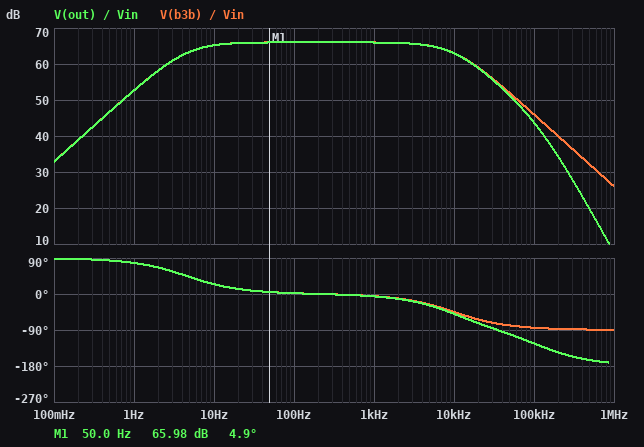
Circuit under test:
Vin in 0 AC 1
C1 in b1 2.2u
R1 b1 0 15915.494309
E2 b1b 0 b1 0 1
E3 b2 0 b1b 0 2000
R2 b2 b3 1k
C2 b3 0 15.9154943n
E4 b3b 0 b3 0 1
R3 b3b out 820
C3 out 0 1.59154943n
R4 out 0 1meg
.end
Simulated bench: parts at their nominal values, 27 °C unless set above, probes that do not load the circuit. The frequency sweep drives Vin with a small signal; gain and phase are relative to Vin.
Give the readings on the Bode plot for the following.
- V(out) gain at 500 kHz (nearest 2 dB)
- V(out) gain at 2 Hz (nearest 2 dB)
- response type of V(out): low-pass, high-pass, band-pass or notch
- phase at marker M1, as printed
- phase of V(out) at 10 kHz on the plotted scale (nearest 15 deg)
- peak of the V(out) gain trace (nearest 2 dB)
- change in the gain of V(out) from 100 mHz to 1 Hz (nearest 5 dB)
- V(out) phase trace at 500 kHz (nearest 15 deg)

20 dB
58 dB
band-pass
4.9 deg
-45 deg
66 dB
20 dB
-165 deg
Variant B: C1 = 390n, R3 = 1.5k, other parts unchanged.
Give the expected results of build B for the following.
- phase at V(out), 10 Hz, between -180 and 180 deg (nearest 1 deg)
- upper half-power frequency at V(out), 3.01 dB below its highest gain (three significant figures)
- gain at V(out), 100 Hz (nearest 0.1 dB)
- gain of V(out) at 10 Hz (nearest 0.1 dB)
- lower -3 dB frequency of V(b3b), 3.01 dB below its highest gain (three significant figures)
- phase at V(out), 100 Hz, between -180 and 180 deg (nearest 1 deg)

69 deg
9.84 kHz
65.7 dB
57.2 dB
25.5 Hz
14 deg
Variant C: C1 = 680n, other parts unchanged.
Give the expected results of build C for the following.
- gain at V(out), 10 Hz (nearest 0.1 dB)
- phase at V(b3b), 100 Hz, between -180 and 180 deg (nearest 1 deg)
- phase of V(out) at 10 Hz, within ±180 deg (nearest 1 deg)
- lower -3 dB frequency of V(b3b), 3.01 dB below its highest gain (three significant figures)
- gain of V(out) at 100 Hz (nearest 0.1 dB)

61.0 dB
8 deg
56 deg
14.7 Hz
65.9 dB
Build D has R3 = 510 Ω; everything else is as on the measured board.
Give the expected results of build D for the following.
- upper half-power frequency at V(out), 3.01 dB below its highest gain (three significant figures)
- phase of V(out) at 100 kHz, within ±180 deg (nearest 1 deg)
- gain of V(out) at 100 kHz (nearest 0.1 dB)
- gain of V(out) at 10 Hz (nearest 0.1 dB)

9.98 kHz
-111 deg
45.0 dB
65.2 dB
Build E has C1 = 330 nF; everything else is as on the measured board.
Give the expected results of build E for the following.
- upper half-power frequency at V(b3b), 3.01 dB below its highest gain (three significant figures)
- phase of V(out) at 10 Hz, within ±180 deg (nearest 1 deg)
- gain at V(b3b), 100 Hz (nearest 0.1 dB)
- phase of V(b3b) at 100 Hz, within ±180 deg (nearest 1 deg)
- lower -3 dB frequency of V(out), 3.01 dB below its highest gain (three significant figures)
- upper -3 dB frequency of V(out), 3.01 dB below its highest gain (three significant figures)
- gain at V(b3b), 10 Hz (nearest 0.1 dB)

10.1 kHz
72 deg
65.6 dB
16 deg
30.1 Hz
9.99 kHz
55.9 dB
